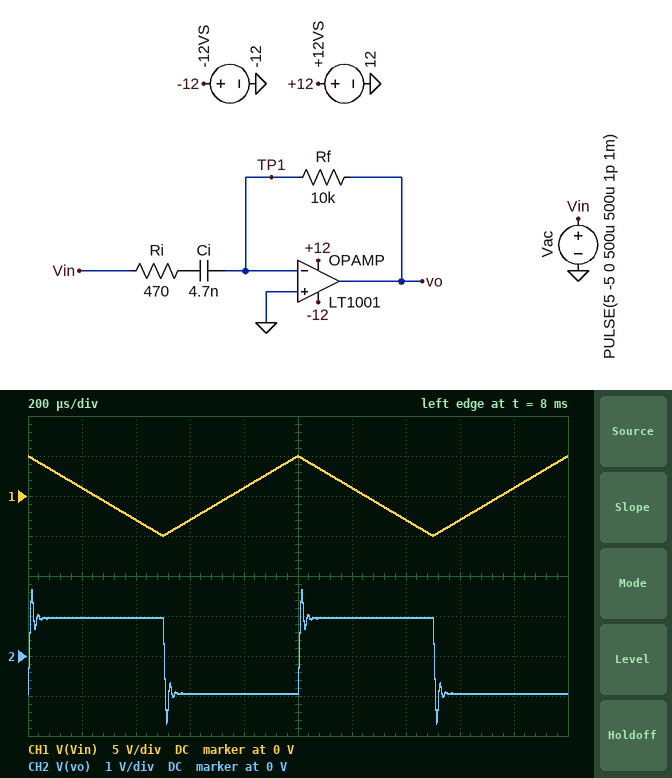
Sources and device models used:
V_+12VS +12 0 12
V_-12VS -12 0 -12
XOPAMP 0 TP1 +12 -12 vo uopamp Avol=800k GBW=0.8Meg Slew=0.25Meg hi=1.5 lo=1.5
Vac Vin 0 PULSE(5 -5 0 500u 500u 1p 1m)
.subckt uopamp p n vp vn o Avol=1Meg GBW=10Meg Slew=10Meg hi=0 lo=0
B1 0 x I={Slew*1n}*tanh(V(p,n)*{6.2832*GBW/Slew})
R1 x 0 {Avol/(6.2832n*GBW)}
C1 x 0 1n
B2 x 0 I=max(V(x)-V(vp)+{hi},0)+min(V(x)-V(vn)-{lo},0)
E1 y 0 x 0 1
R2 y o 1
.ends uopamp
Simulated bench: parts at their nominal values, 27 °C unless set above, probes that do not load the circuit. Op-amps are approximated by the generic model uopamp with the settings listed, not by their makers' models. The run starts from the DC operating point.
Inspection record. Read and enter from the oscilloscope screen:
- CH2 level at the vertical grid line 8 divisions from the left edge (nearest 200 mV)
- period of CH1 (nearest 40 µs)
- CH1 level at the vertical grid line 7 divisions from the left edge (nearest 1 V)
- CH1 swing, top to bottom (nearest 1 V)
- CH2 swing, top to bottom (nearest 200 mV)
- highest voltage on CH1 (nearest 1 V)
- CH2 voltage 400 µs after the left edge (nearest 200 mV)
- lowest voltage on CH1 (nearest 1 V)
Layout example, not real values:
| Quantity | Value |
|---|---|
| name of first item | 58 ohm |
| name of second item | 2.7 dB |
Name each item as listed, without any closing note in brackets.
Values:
| Quantity | Value |
|---|---|
| CH2 level at the vertical grid line 8 divisions from the left edge | -1.0 V |
| period of CH1 | 1.00 ms |
| CH1 level at the vertical grid line 7 divisions from the left edge | -3 V |
| CH1 swing, top to bottom | 10 V |
| CH2 swing, top to bottom | 3.4 V |
| highest voltage on CH1 | 5 V |
| CH2 voltage 400 µs after the left edge | 1.0 V |
| lowest voltage on CH1 | -5 V |
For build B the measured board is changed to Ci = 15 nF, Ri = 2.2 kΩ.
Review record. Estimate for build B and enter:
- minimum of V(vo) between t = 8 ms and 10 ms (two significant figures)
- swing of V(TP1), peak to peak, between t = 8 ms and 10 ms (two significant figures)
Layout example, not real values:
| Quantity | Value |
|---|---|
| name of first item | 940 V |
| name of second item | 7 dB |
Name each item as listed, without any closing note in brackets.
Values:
| Quantity | Value |
|---|---|
| minimum of V(vo) between t = 8 ms and 10 ms | -3.0 V |
| swing of V(TP1), peak to peak, between t = 8 ms and 10 ms | 78 mV |
